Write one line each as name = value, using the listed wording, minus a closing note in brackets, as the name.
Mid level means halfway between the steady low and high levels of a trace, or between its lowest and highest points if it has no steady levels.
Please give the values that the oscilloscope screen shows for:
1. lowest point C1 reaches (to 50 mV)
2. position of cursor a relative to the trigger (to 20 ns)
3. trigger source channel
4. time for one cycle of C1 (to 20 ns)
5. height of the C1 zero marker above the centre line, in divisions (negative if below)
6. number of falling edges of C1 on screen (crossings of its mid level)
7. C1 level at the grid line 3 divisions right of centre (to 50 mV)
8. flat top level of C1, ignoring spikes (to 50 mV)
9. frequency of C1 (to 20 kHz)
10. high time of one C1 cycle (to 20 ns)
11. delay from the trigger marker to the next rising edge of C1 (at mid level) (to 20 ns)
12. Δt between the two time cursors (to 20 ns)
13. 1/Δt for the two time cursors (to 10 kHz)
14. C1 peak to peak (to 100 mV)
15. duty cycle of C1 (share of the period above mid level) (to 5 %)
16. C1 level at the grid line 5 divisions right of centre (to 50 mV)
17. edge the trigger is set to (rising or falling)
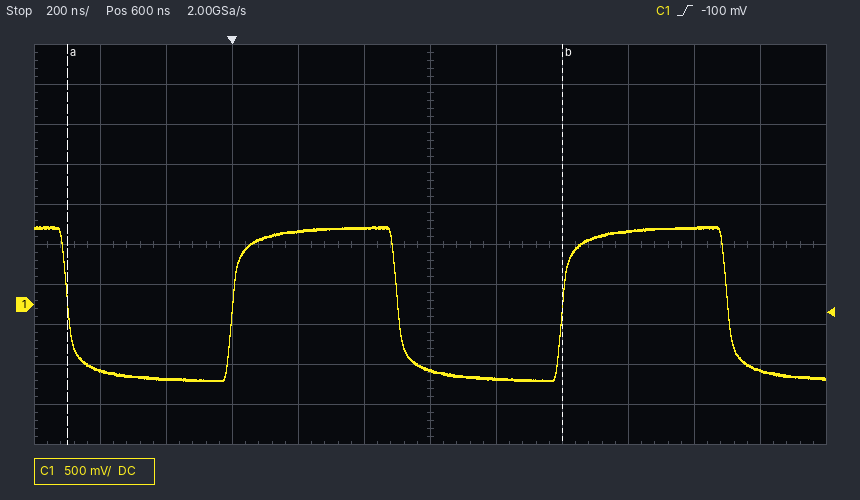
lowest point C1 reaches = -950 mV
position of cursor a relative to the trigger = -500 ns
trigger source channel = C1
time for one cycle of C1 = 1.00 µs
height of the C1 zero marker above the centre line, in divisions = -1.5 div
number of falling edges of C1 on screen = 3
C1 level at the grid line 3 divisions right of centre = 900 mV
flat top level of C1, ignoring spikes = 950 mV
frequency of C1 = 1.00 MHz
high time of one C1 cycle = 500 ns
delay from the trigger marker to the next rising edge of C1 (at mid level) = 1.00 µs
Δt between the two time cursors = 1.50 µs
1/Δt for the two time cursors = 670 kHz
C1 peak to peak = 1.90 V
duty cycle of C1 (share of the period above mid level) = 50 %
C1 level at the grid line 5 divisions right of centre = -800 mV
edge the trigger is set to = rising
